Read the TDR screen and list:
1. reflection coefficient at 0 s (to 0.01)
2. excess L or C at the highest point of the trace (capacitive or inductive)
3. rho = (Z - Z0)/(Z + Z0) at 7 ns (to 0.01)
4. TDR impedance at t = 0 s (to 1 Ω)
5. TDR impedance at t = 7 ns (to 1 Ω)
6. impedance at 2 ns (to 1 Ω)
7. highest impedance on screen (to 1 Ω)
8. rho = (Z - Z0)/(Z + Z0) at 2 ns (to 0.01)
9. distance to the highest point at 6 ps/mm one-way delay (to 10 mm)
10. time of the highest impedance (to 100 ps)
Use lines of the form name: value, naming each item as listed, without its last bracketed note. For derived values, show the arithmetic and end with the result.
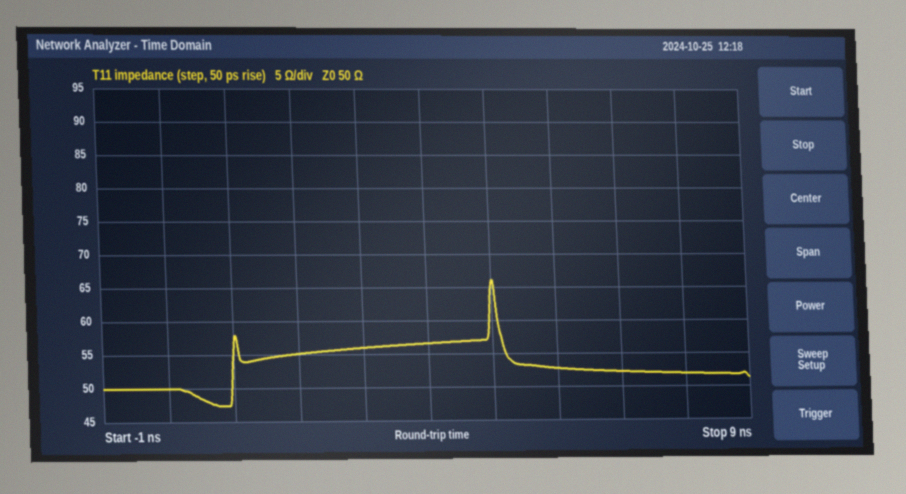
reflection coefficient at 0 s: (50 − 50)/(50 + 50) ≈ 0.00
excess L or C at the highest point of the trace: inductive
rho = (Z - Z0)/(Z + Z0) at 7 ns: (52 − 50)/(52 + 50) ≈ +0.02
TDR impedance at t = 0 s: 50 Ω
TDR impedance at t = 7 ns: 52 Ω
impedance at 2 ns: 55 Ω
highest impedance on screen: 66 Ω
rho = (Z - Z0)/(Z + Z0) at 2 ns: (55 − 50)/(55 + 50) ≈ +0.05
distance to the highest point at 6 ps/mm one-way delay: 5.0 ns / 2 / 6 ps/mm ≈ 417 mm, so 420 mm to the nearest 10 mm
time of the highest impedance: 5.0 ns
